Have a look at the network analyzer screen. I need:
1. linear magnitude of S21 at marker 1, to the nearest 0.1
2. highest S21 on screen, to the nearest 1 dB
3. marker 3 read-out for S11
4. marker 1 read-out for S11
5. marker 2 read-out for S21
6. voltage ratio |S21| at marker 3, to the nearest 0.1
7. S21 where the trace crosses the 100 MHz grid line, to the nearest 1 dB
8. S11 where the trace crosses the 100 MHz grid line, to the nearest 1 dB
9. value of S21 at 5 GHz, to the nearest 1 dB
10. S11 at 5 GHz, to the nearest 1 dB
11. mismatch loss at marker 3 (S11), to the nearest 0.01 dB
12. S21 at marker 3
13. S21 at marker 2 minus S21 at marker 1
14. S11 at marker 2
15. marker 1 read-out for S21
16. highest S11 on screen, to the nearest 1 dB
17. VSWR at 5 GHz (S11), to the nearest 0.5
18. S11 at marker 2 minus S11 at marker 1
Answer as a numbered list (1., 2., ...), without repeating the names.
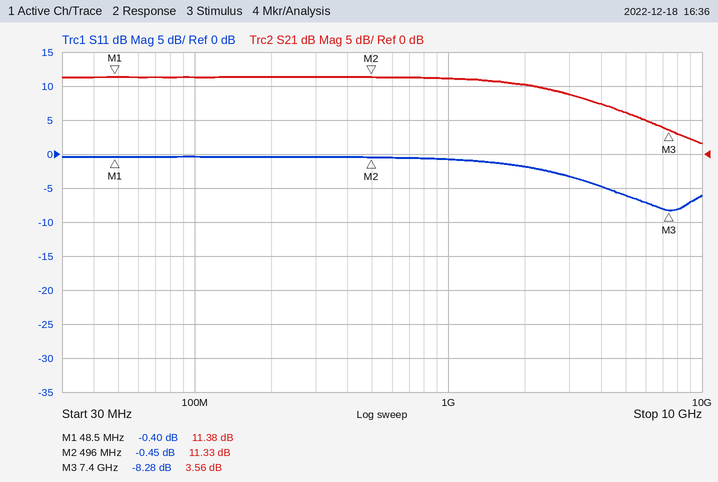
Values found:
1. 3.7
2. 11 dB
3. -8.28 dB
4. -0.40 dB
5. 11.33 dB
6. 1.5
7. 11 dB
8. 0 dB
9. 6 dB
10. -6 dB
11. 0.70 dB
12. 3.56 dB
13. -0.05 dB
14. -0.45 dB
15. 11.38 dB
16. 0 dB
17. 3.0
18. -0.05 dB
